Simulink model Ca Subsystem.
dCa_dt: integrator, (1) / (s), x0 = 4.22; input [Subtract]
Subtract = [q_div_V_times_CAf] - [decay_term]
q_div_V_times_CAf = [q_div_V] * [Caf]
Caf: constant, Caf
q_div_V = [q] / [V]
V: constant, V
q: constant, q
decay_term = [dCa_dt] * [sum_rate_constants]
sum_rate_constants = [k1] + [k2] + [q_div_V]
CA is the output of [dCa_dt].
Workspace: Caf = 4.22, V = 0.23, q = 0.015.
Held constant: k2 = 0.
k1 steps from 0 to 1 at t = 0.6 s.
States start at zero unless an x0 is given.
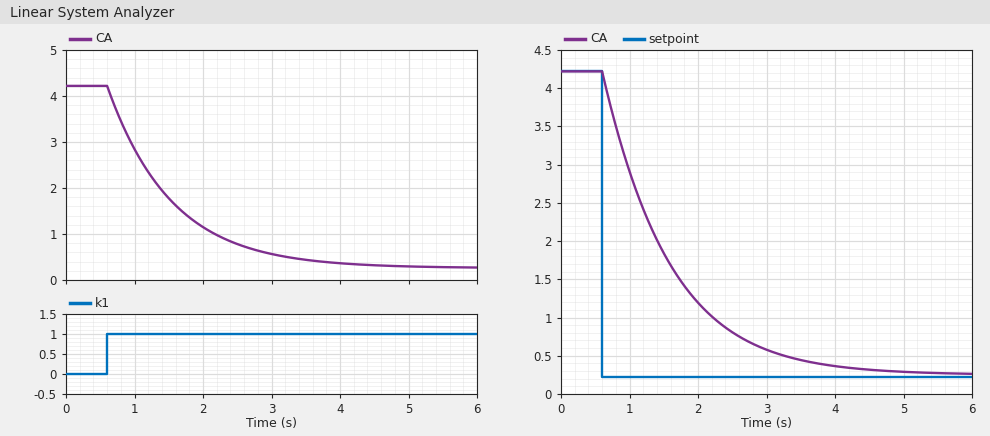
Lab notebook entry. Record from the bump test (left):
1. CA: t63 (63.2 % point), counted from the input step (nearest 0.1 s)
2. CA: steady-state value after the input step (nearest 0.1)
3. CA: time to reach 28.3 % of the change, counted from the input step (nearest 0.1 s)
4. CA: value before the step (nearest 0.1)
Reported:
0.9 s
0.3
0.3 s
4.2
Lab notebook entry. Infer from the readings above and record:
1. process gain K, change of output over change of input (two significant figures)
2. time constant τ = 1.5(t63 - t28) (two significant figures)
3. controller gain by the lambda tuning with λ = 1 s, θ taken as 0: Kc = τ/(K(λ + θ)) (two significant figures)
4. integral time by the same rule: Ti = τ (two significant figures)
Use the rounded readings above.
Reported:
-3.9
0.90 s
-0.23
0.90 s
